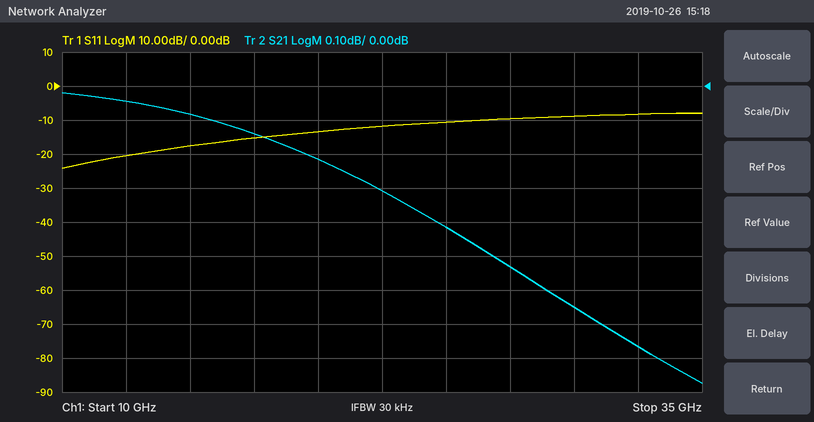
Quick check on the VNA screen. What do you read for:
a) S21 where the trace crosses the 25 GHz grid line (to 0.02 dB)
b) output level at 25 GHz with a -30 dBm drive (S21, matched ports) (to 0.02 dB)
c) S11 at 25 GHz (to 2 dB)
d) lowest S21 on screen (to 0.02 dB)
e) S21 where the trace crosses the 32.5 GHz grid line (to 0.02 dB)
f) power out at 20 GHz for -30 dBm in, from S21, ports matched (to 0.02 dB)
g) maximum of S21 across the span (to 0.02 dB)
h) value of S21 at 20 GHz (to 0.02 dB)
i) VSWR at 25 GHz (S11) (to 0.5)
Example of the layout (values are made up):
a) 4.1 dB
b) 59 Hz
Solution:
a) -0.42 dB
b) -30.42 dBm
c) -10 dB
d) -0.88 dB
e) -0.76 dB
f) -30.22 dBm
g) -0.02 dB
h) -0.22 dB
i) 2.0
